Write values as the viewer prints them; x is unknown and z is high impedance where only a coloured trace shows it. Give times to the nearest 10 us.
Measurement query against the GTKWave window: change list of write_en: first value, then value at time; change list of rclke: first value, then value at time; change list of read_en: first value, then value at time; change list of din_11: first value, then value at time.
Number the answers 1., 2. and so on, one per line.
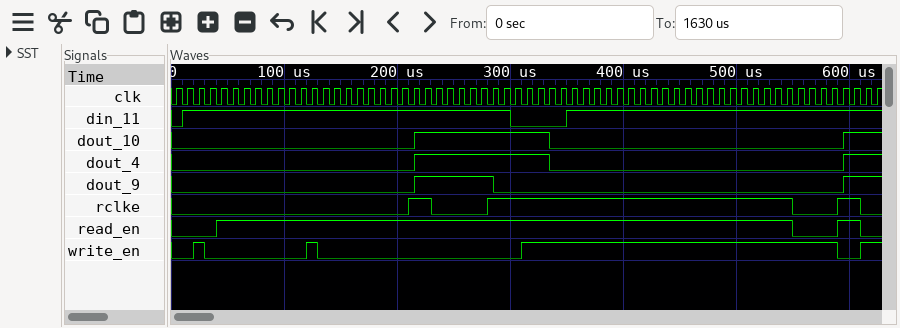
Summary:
1. 0, 1 at 20 us, 0 at 30 us, 1 at 120 us, 0 at 130 us, 1 at 310 us, 0 at 590 us, 1 at 610 us
2. 0, 1 at 210 us, 0 at 230 us, 1 at 280 us, 0 at 550 us, 1 at 590 us, 0 at 610 us
3. 0, 1 at 40 us, 0 at 550 us, 1 at 590 us, 0 at 610 us
4. 0, 1 at 10 us, 0 at 300 us, 1 at 350 us
